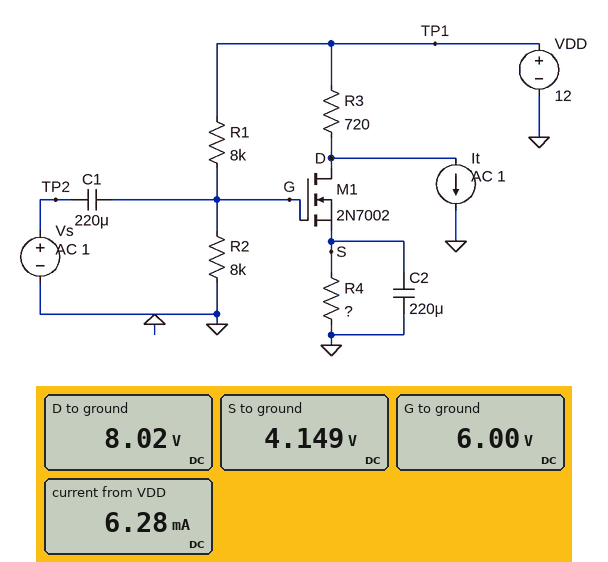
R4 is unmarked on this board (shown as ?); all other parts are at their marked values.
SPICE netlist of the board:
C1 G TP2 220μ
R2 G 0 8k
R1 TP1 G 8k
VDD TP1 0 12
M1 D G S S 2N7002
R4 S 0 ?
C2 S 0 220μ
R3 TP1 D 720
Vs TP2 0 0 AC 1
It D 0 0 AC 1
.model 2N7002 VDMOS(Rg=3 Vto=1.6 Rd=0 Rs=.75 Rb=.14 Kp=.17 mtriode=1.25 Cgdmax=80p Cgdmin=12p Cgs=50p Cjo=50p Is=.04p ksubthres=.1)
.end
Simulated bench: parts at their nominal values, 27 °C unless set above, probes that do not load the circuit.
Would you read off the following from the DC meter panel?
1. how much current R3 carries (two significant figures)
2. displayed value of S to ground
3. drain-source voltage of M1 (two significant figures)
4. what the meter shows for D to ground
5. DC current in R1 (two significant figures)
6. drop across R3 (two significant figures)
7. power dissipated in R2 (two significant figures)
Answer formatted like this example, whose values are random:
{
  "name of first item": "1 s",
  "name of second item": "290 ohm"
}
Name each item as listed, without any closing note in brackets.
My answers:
{
  "how much current R3 carries": "5.5 mA",
  "displayed value of S to ground": "4.149 V",
  "drain-source voltage of M1": "3.9 V",
  "what the meter shows for D to ground": "8.02 V",
  "DC current in R1": "750 µA",
  "drop across R3": "4.0 V",
  "power dissipated in R2": "4.5 mW"
}
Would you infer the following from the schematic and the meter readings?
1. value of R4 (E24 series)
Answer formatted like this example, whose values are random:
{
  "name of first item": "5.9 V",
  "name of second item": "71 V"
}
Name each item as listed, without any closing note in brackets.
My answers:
{
  "value of R4": "750 Ω"
}
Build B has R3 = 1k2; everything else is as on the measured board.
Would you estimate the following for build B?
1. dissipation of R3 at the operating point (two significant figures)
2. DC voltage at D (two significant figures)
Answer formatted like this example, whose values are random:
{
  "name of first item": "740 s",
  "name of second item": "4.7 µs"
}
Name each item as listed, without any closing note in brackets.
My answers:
{
  "dissipation of R3 at the operating point": "37 mW",
  "DC voltage at D": "5.4 V"
}
